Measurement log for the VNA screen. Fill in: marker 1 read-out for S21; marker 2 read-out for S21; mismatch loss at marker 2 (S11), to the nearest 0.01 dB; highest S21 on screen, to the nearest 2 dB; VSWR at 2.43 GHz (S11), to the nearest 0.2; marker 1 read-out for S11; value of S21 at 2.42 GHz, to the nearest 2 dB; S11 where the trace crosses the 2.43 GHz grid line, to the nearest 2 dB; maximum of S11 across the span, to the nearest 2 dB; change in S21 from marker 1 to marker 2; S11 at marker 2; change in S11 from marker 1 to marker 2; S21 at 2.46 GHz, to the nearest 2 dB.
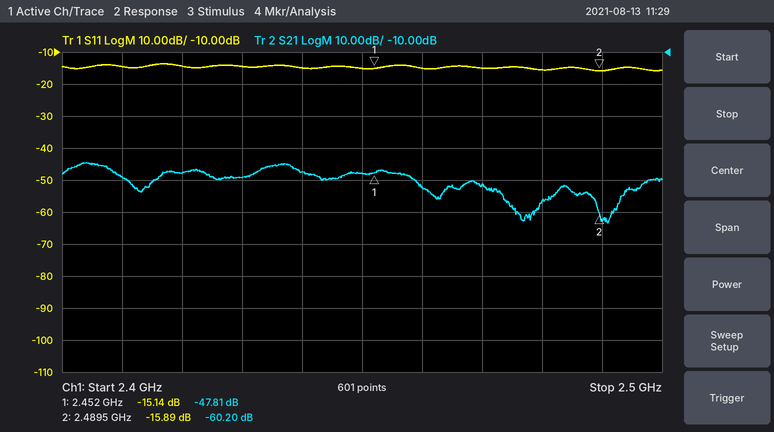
-47.81 dB
-60.20 dB
0.11 dB
-44 dB
1.4
-15.14 dB
-48 dB
-14 dB
-14 dB
-12.39 dB
-15.89 dB
-0.75 dB
-52 dB
